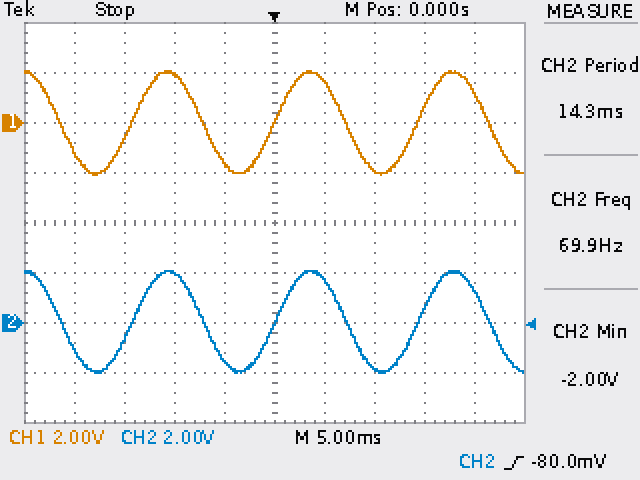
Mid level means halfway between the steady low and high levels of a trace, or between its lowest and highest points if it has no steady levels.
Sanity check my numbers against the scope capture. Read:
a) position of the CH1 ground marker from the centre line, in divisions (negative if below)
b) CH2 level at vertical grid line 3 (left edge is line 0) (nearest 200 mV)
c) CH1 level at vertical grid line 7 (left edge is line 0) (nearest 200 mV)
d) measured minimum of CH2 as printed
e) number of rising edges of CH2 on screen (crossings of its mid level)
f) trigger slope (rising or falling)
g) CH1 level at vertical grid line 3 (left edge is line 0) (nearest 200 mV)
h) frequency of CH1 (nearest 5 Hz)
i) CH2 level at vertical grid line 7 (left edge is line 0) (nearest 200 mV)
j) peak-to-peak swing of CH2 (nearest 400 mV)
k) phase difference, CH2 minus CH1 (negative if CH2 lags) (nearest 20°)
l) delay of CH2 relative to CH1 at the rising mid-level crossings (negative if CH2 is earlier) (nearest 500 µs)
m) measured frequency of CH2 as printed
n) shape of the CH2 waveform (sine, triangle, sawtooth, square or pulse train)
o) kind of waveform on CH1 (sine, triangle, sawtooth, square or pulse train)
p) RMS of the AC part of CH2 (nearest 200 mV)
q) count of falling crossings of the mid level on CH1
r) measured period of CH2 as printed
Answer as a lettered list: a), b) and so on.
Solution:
a) +2.0 div
b) 2.0 V
c) -1.8 V
d) -2.00 V
e) 3
f) rising
g) 2.0 V
h) 70 Hz
i) -1.8 V
j) 4.0 V
k) 0°
l) 0.0 ms
m) 69.9 Hz
n) sine
o) sine
p) 1.4 V
q) 4
r) 14.3 ms
